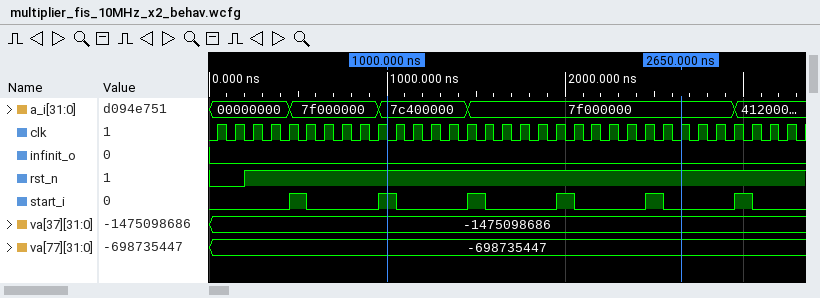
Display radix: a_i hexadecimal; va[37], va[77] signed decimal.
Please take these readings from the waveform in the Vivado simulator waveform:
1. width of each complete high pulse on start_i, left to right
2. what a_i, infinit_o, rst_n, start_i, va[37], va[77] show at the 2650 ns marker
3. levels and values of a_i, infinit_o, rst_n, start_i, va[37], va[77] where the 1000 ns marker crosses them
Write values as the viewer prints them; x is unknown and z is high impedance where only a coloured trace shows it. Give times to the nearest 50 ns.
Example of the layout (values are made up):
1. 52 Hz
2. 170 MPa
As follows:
1. 100 ns, 100 ns, 100 ns, 100 ns, 100 ns, 100 ns
2. a_i=7f000000, infinit_o=0, rst_n=1, start_i=0, va[37]=-1475098686, va[77]=-698735447
3. a_i=7c400000, infinit_o=0, rst_n=1, start_i=1, va[37]=-1475098686, va[77]=-698735447
